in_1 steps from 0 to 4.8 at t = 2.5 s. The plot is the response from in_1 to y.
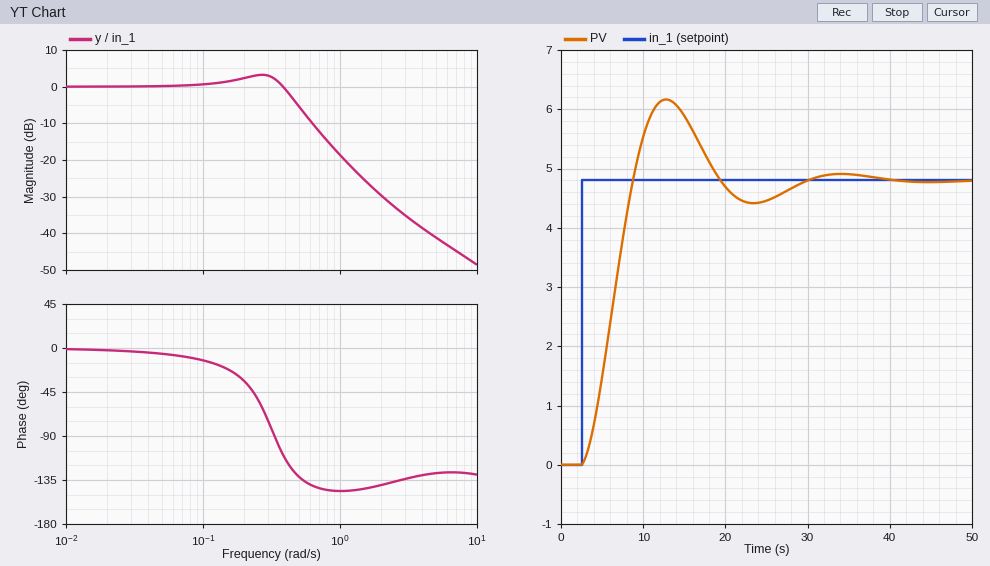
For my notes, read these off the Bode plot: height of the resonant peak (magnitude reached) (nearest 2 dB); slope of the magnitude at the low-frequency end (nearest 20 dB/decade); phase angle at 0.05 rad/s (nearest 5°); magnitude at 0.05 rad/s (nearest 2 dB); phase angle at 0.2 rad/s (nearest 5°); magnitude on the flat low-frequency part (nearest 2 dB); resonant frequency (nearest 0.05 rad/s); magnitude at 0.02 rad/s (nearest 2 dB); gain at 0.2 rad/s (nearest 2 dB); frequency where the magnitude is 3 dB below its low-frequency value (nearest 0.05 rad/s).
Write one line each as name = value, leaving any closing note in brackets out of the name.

height of the resonant peak (magnitude reached) = 4 dB
slope of the magnitude at the low-frequency end = 0 dB/decade
phase angle at 0.05 rad/s = -5°
magnitude at 0.05 rad/s = 0 dB
phase angle at 0.2 rad/s = -35°
magnitude on the flat low-frequency part = 0 dB
resonant frequency = 0.25 rad/s
magnitude at 0.02 rad/s = 0 dB
gain at 0.2 rad/s = 2 dB
frequency where the magnitude is 3 dB below its low-frequency value = 0.45 rad/s
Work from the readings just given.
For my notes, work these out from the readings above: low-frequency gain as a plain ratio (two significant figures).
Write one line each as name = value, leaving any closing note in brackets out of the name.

low-frequency gain as a plain ratio = 1.0
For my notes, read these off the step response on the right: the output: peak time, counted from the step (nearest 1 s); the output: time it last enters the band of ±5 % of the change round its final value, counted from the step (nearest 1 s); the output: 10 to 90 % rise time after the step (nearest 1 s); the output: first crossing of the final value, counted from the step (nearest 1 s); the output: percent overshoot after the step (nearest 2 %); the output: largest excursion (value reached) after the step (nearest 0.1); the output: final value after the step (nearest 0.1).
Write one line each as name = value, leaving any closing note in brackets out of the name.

the output: peak time, counted from the step = 10 s
the output: time it last enters the band of ±5 % of the change round its final value, counted from the step = 24 s
the output: 10 to 90 % rise time after the step = 4 s
the output: first crossing of the final value, counted from the step = 6 s
the output: percent overshoot after the step = 28 %
the output: largest excursion (value reached) after the step = 6.2
the output: final value after the step = 4.8
